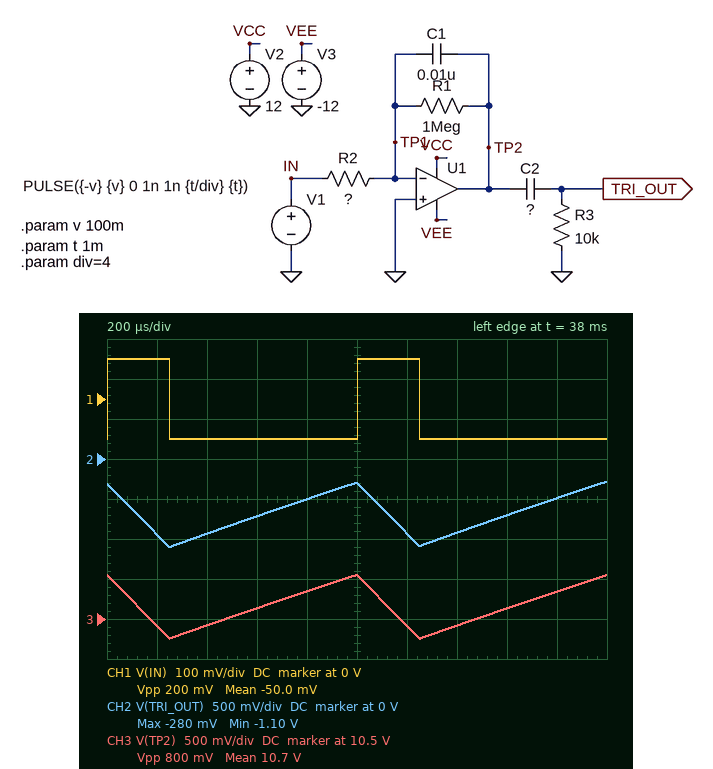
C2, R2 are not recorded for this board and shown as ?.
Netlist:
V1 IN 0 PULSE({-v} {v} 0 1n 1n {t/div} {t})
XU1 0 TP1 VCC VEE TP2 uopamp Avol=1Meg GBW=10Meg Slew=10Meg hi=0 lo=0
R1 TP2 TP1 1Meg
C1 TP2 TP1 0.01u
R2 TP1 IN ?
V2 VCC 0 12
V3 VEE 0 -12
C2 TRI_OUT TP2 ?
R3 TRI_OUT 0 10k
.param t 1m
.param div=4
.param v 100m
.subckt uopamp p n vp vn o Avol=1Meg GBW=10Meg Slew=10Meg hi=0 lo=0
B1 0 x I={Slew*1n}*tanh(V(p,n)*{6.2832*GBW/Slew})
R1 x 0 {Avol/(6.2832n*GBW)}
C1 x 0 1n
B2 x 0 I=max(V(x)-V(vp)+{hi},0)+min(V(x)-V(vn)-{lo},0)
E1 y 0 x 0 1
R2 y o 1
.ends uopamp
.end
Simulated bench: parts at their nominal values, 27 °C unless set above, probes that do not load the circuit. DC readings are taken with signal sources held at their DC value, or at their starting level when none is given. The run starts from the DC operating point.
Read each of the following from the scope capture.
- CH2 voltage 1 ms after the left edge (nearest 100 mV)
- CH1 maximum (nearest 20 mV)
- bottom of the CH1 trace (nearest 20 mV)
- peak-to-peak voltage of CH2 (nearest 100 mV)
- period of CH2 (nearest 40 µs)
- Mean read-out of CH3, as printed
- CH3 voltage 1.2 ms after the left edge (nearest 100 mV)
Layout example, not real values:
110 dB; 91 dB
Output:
-300 mV; 100 mV; -100 mV; 800 mV; 1.00 ms; 10.7 V; 10.4 V
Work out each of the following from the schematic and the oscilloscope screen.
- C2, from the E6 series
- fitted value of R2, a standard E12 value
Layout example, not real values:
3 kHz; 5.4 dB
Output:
4.7 µF; 4.7 kΩ
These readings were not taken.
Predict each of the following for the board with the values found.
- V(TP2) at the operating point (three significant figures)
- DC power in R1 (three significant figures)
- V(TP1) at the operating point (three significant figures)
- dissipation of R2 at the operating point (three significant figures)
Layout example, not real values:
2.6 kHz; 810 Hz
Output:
12.0 V; 145 µW; -43.4 mV; 682 nW
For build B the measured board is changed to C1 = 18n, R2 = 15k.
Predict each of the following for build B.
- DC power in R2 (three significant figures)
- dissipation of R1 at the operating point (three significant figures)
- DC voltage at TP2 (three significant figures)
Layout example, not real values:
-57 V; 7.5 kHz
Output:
667 nW; 44.4 µW; 6.67 V
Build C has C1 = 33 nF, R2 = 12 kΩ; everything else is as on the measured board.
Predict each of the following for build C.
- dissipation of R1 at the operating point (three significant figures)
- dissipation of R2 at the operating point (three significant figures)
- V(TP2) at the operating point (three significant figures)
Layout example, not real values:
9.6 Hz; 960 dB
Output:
69.4 µW; 833 nW; 8.33 V
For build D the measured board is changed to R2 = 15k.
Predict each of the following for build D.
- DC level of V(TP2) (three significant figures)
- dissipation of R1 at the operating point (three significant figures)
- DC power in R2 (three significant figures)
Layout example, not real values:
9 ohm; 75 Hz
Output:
6.67 V; 44.4 µW; 667 nW
